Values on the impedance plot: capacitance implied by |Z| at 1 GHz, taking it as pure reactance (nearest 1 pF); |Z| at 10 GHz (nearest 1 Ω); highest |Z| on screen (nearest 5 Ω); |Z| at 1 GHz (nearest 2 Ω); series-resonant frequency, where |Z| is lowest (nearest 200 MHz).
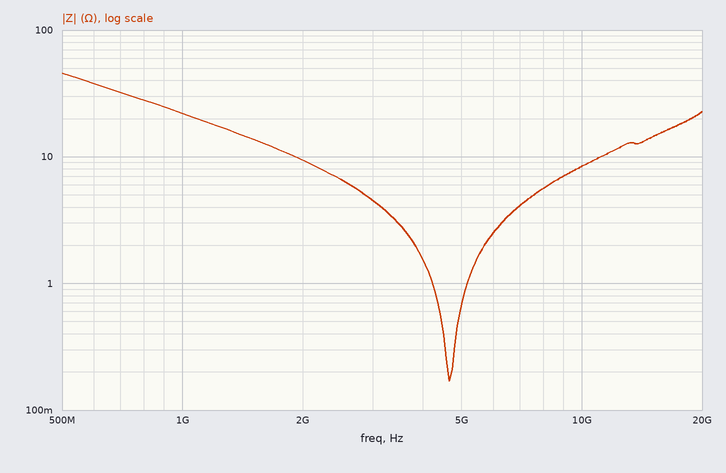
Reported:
7 pF
8 Ω
45 Ω
22 Ω
4.6 GHz
